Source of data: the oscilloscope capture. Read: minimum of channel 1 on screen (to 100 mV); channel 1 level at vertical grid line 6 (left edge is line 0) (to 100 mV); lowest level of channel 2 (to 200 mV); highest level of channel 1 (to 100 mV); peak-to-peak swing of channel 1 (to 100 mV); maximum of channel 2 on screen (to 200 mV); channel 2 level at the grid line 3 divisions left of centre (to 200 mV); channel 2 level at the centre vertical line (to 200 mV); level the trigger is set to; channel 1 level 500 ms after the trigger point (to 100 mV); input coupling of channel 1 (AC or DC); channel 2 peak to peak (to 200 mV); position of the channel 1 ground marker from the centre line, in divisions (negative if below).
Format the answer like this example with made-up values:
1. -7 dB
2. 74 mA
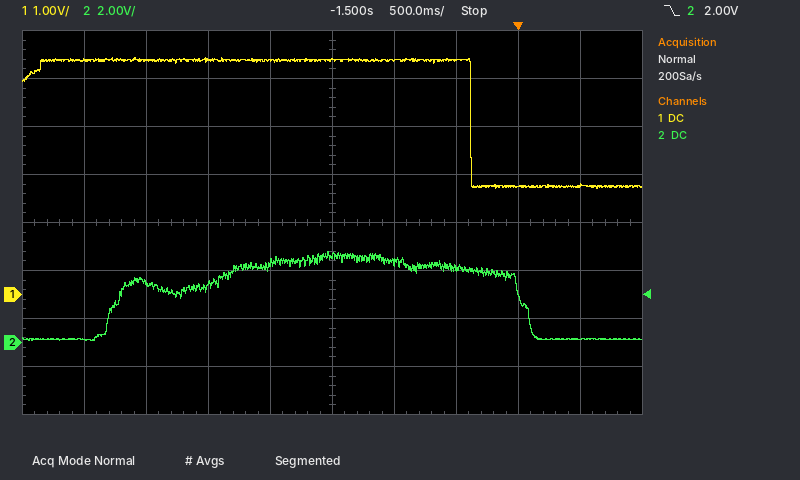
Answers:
1. 2.2 V
2. 4.9 V
3. 0.0 V
4. 4.9 V
5. 2.7 V
6. 3.8 V
7. 2.4 V
8. 3.6 V
9. 2.00 V
10. 2.3 V
11. DC
12. 3.8 V
13. -1.5 div
